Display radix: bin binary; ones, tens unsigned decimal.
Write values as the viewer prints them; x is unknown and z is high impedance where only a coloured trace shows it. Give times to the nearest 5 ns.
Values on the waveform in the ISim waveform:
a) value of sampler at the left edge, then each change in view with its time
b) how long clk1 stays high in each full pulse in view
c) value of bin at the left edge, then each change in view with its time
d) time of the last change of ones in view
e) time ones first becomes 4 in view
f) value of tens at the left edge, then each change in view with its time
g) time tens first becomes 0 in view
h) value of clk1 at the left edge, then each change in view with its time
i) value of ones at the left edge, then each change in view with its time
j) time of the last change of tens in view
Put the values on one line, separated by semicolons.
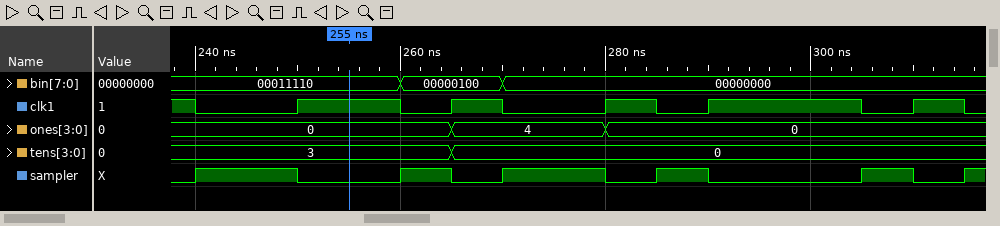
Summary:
0, 1 at 240 ns, 0 at 250 ns, 1 at 260 ns, 0 at 265 ns, 1 at 270 ns, 0 at 280 ns, 1 at 285 ns, 0 at 290 ns, 1 at 305 ns, 0 at 310 ns, 1 at 315 ns; 10 ns, 5 ns, 5 ns, 15 ns, 5 ns; 00011110, 00000100 at 260 ns, 00000000 at 270 ns; 280 ns; 265 ns; 3, 0 at 265 ns; 265 ns; 1, 0 at 240 ns, 1 at 250 ns, 0 at 260 ns, 1 at 265 ns, 0 at 270 ns, 1 at 280 ns, 0 at 285 ns, 1 at 290 ns, 0 at 305 ns, 1 at 310 ns, 0 at 315 ns; 0, 4 at 265 ns, 0 at 280 ns; 265 ns
